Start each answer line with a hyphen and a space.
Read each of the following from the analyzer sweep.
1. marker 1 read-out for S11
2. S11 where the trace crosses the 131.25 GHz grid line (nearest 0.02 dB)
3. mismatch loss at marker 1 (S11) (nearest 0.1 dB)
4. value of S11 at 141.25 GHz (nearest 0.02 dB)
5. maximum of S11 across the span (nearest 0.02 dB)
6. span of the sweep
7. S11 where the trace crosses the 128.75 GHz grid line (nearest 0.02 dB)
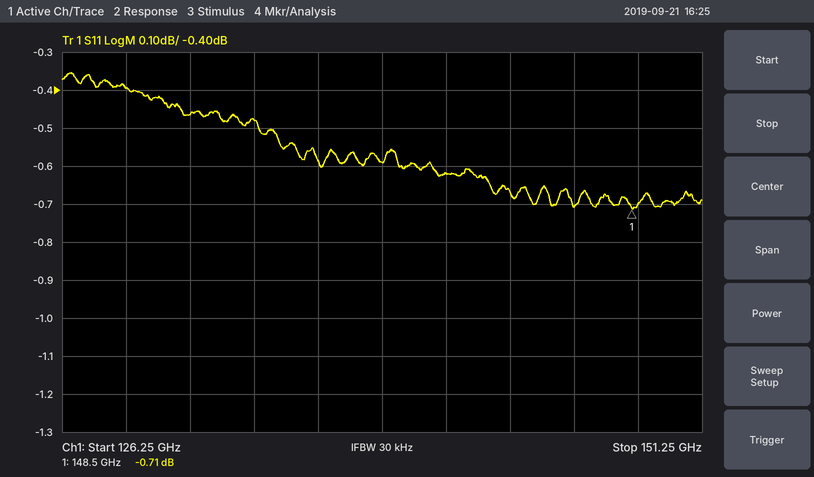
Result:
- -0.71 dB
- -0.46 dB
- 8.2 dB
- -0.62 dB
- -0.36 dB
- 25 GHz
- -0.40 dB
